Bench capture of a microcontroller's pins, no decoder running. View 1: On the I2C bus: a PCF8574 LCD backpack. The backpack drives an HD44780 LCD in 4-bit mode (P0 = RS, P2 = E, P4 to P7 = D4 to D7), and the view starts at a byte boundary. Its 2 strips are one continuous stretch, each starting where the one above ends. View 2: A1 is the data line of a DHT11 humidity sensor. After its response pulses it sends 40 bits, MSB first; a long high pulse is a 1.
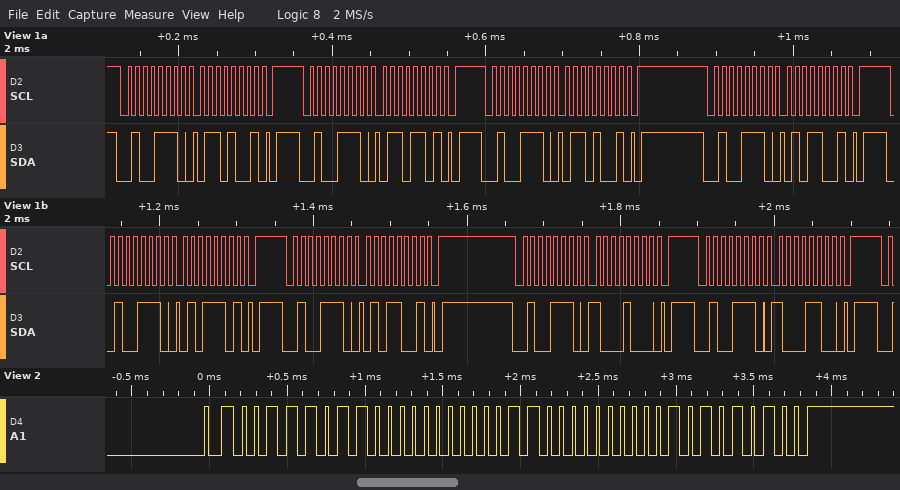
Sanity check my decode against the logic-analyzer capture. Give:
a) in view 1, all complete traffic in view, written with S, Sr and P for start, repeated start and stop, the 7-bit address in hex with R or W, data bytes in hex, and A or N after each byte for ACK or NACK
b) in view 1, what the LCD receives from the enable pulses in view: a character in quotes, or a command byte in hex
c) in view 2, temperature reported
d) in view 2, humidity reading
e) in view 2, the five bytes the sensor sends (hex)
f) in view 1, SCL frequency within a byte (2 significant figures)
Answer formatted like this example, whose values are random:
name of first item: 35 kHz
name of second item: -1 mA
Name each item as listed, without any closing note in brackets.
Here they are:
in view 1, all complete traffic in view, written with S, Sr and P for start, repeated start and stop, the 7-bit address in hex with R or W, data bytes in hex, and A or N after each byte for ACK or NACK: S 27W A 69 A P S 27W A 6D A P S 27W A 69 A P S 27W A 59 A P S 27W A 5D A P S 27W A 59 A P S 27W A 88 A P S 27W A 8C A P
in view 1, what the LCD receives from the enable pulses in view: a character in quotes, or a command byte in hex: 'e'
in view 2, temperature reported: 24.1 °C
in view 2, humidity reading: 59 %
in view 2, the five bytes the sensor sends: 3B 00 18 01 54
in view 1, SCL frequency within a byte: 100 kHz
